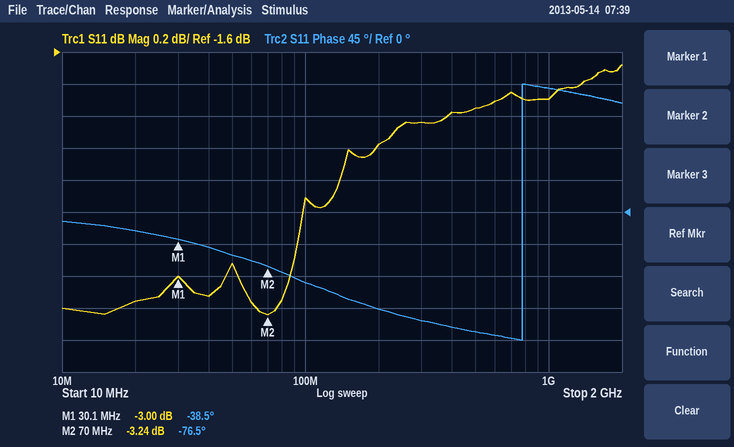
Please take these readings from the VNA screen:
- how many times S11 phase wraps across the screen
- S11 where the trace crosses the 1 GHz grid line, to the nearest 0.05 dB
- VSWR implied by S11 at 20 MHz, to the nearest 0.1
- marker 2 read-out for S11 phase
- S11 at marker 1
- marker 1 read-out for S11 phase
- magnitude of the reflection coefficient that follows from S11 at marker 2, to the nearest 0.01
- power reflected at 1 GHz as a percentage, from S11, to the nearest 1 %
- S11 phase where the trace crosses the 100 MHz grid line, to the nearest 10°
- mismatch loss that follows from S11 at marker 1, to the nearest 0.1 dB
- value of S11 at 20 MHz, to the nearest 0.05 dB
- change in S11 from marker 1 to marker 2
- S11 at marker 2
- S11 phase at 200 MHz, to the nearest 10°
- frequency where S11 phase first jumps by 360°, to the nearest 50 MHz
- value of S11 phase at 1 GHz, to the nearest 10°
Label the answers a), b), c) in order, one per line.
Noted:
a) 1
b) -1.90 dB
c) 5.6
d) -76.5°
e) -3.00 dB
f) -38.5°
g) 0.69
h) 65 %
i) -100°
j) 3.0 dB
k) -3.15 dB
l) -0.24 dB
m) -3.24 dB
n) -140°
o) 800 MHz
p) 170°
